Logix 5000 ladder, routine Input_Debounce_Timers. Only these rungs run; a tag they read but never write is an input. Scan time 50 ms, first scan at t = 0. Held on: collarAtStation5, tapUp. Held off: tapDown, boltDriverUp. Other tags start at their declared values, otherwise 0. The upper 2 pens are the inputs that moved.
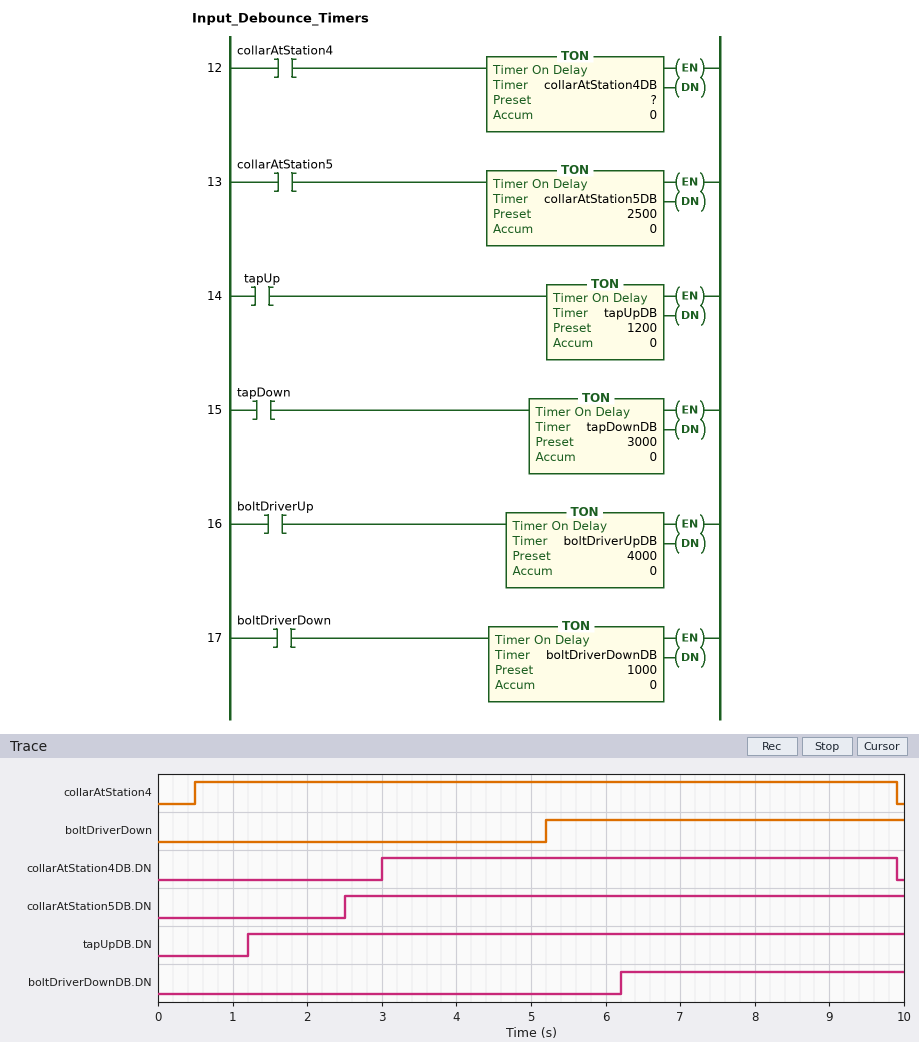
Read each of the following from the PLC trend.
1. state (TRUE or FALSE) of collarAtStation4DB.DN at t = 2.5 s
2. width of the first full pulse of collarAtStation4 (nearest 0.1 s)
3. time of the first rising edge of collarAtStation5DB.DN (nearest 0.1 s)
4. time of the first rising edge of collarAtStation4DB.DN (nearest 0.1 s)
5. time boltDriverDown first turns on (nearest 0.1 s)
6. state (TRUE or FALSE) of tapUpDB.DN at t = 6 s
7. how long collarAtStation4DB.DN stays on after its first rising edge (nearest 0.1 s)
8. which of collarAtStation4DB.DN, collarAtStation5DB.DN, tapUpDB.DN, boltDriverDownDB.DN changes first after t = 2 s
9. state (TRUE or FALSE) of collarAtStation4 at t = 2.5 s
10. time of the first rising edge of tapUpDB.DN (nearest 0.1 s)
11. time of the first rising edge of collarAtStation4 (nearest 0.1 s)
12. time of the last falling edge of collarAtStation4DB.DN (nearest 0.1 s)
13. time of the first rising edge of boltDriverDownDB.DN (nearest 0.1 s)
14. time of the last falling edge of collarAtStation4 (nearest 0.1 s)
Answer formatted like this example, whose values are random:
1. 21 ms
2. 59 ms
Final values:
1. FALSE
2. 9.4 s
3. 2.5 s
4. 3.0 s
5. 5.2 s
6. TRUE
7. 6.9 s
8. collarAtStation5DB.DN
9. TRUE
10. 1.2 s
11. 0.5 s
12. 9.9 s
13. 6.2 s
14. 9.9 s
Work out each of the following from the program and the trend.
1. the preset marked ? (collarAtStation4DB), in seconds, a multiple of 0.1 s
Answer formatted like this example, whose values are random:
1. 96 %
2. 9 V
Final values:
1. 2.5 s
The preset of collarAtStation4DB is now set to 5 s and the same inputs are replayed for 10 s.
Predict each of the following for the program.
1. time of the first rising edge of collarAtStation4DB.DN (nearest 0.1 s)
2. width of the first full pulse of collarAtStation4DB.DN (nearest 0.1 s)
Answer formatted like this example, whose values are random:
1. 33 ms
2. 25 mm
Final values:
1. 5.5 s
2. 4.4 s
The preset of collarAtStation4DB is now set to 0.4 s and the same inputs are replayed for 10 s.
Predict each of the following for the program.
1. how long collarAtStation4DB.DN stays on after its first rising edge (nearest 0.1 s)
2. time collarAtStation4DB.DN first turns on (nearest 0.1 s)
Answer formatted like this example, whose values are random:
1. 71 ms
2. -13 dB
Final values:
1. 9.0 s
2. 0.9 s
